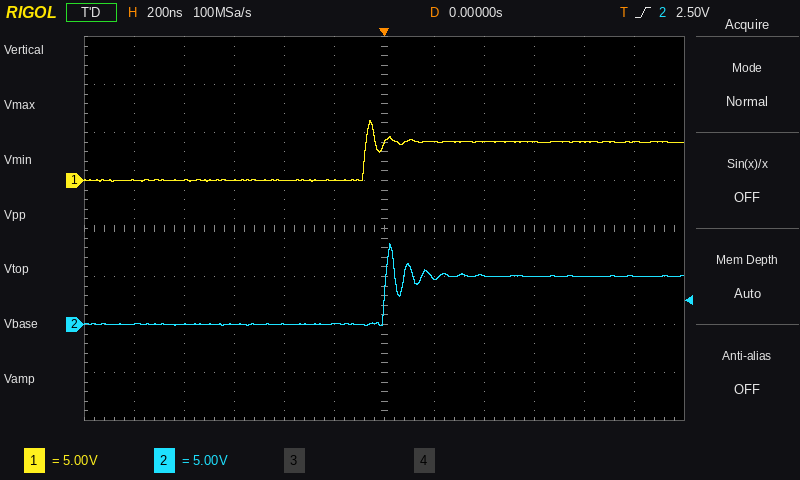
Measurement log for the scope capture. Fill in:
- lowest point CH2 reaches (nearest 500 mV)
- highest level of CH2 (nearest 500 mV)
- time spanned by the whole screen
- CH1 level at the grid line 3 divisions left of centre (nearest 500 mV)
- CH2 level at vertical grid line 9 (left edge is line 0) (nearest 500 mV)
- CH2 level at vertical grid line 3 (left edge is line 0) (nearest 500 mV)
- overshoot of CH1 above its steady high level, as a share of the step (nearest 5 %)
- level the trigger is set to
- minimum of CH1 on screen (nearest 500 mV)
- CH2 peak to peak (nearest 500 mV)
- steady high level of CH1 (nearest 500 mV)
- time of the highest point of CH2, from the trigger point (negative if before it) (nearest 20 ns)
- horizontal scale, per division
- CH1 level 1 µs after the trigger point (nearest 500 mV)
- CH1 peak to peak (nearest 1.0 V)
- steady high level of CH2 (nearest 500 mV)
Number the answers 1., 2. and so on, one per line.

1. 0.0 V
2. 8.5 V
3. 2.4 µs
4. 0.0 V
5. 5.0 V
6. 0.0 V
7. 55 %
8. 2.50 V
9. 0.0 V
10. 8.5 V
11. 4.0 V
12. +20 ns
13. 200 ns
14. 4.0 V
15. 6.0 V
16. 5.0 V
